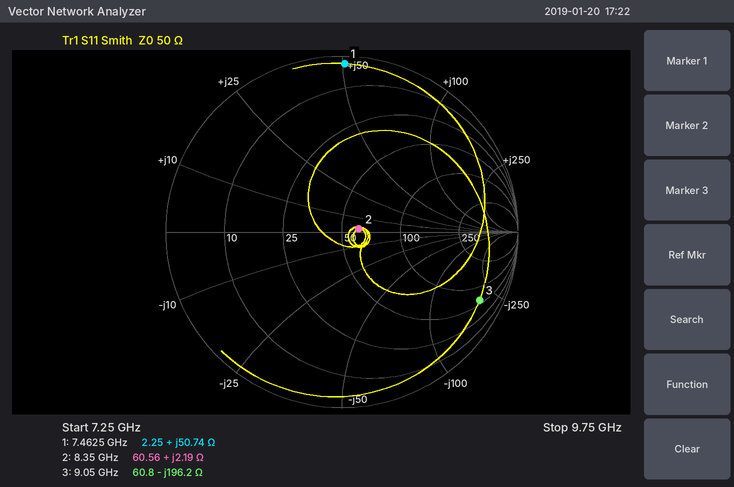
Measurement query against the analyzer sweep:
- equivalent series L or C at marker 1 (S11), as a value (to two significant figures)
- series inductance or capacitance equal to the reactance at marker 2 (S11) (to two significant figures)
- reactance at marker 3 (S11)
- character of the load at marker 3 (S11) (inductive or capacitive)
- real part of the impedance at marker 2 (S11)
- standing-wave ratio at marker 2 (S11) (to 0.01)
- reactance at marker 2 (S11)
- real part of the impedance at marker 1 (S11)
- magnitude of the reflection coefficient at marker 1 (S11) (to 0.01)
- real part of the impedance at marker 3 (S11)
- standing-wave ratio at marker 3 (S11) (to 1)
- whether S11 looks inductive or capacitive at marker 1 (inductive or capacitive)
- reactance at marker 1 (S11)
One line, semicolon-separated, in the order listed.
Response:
1.1 nH; 42 pH; -196.2 Ω; capacitive; 60.56 Ω; 1.22; +2.19 Ω; 2.25 Ω; 0.96; 60.8 Ω; 15; inductive; +50.74 Ω
